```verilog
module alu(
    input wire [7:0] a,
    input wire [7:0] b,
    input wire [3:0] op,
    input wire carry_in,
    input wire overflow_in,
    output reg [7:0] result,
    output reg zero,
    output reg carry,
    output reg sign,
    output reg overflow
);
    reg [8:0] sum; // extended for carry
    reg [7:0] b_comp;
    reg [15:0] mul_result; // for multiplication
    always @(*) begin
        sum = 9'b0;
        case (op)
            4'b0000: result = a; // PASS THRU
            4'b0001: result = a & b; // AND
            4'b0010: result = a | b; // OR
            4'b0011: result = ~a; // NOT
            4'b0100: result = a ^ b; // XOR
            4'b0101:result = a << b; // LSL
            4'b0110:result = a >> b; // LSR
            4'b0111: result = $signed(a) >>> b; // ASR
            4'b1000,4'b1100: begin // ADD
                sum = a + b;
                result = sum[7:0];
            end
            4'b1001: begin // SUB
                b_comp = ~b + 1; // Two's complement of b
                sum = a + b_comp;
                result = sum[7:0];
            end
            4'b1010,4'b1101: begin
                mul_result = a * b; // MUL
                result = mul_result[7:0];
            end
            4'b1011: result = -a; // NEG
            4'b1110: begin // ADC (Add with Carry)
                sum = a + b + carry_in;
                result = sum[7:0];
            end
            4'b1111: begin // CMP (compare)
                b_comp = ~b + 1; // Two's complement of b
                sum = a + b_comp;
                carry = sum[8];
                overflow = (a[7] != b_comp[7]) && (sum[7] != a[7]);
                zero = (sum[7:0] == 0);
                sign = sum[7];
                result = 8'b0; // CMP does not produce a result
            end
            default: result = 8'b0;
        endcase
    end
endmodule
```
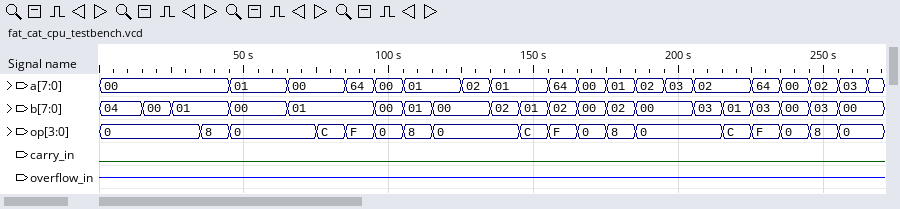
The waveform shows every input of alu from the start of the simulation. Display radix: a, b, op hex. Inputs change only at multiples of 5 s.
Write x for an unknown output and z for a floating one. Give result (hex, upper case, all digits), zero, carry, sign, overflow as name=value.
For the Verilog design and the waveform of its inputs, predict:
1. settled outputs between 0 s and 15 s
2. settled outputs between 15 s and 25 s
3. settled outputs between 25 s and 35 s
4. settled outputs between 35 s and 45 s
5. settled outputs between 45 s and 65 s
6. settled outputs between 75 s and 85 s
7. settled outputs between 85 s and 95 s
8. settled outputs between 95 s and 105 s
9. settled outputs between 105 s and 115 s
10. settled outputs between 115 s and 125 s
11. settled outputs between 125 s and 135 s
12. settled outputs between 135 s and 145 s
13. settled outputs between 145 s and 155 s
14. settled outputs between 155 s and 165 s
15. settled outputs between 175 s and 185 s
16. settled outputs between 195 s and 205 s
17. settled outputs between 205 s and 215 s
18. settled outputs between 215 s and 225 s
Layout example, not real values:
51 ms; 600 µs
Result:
result=00, zero=x, carry=x, sign=x, overflow=x; result=00, zero=x, carry=x, sign=x, overflow=x; result=00, zero=x, carry=x, sign=x, overflow=x; result=01, zero=x, carry=x, sign=x, overflow=x; result=01, zero=x, carry=x, sign=x, overflow=x; result=01, zero=x, carry=x, sign=x, overflow=x; result=00, zero=0, carry=1, sign=0, overflow=0; result=00, zero=0, carry=1, sign=0, overflow=0; result=02, zero=0, carry=1, sign=0, overflow=0; result=01, zero=0, carry=1, sign=0, overflow=0; result=02, zero=0, carry=1, sign=0, overflow=0; result=01, zero=0, carry=1, sign=0, overflow=0; result=02, zero=0, carry=1, sign=0, overflow=0; result=00, zero=0, carry=1, sign=0, overflow=0; result=03, zero=0, carry=1, sign=0, overflow=0; result=03, zero=0, carry=1, sign=0, overflow=0; result=02, zero=0, carry=1, sign=0, overflow=0; result=03, zero=0, carry=1, sign=0, overflow=0
